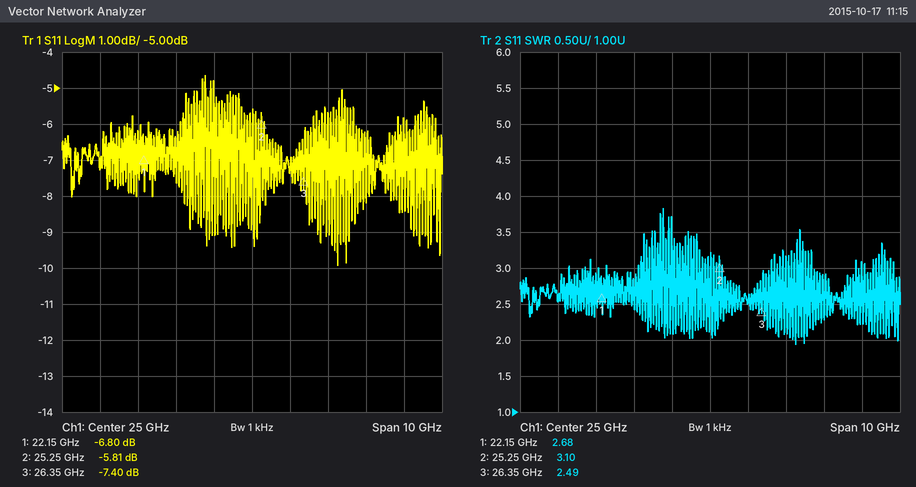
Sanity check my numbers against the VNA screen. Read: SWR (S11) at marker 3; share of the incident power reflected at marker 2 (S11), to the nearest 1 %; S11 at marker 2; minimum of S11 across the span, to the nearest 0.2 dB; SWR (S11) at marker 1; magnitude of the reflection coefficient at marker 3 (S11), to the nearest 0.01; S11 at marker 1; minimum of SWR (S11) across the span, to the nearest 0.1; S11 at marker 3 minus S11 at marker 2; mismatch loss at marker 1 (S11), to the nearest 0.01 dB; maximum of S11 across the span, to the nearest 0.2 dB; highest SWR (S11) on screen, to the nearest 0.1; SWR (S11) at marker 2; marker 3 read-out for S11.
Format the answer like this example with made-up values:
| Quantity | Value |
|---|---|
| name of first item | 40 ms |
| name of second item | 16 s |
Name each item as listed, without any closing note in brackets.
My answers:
| Quantity | Value |
|---|---|
| SWR (S11) at marker 3 | 2.49 |
| share of the incident power reflected at marker 2 (S11), to the nearest 1 % | 26 % |
| S11 at marker 2 | -5.81 dB |
| minimum of S11 across the span, to the nearest 0.2 dB | -10.0 dB |
| SWR (S11) at marker 1 | 2.68 |
| magnitude of the reflection coefficient at marker 3 (S11), to the nearest 0.01 | 0.43 |
| S11 at marker 1 | -6.80 dB |
| minimum of SWR (S11) across the span, to the nearest 0.1 | 1.9 |
| S11 at marker 3 minus S11 at marker 2 | -1.59 dB |
| mismatch loss at marker 1 (S11), to the nearest 0.01 dB | 1.02 dB |
| maximum of S11 across the span, to the nearest 0.2 dB | -4.6 dB |
| highest SWR (S11) on screen, to the nearest 0.1 | 3.8 |
| SWR (S11) at marker 2 | 3.10 |
| marker 3 read-out for S11 | -7.40 dB |
